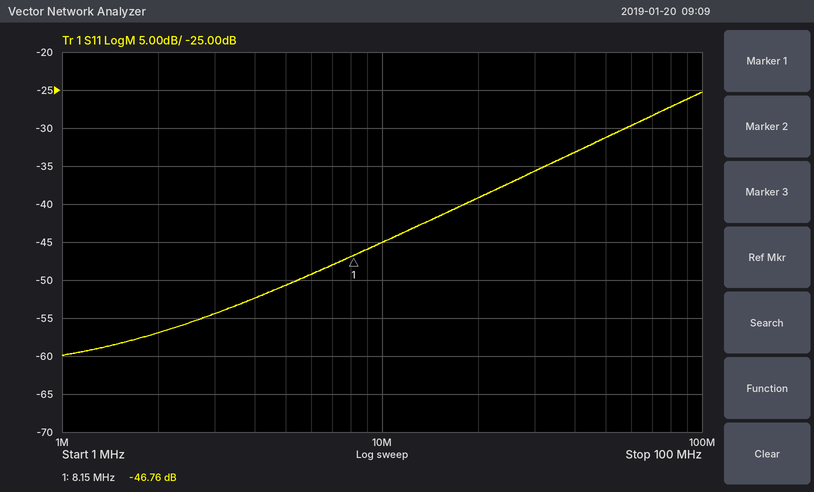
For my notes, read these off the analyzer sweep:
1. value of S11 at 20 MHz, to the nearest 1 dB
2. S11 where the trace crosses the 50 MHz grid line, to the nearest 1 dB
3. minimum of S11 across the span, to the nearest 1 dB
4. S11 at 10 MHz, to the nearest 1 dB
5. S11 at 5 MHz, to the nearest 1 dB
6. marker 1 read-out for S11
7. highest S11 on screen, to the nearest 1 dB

-39 dB
-31 dB
-60 dB
-45 dB
-51 dB
-46.76 dB
-25 dB
